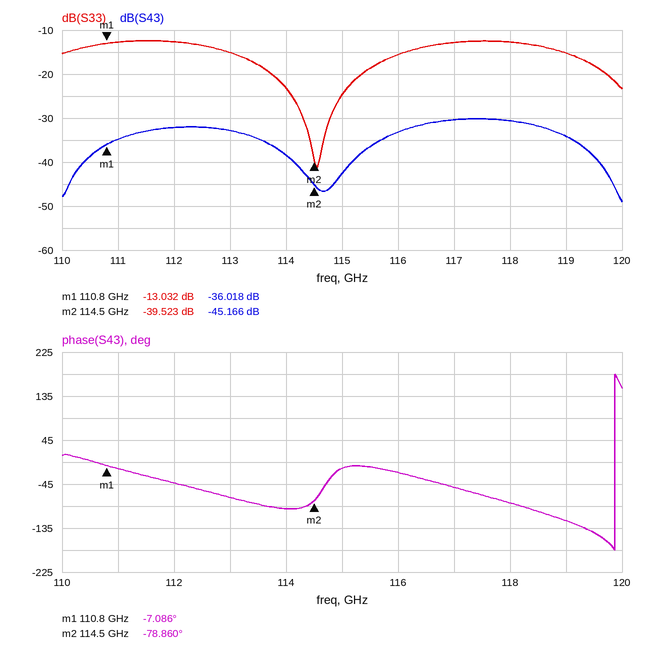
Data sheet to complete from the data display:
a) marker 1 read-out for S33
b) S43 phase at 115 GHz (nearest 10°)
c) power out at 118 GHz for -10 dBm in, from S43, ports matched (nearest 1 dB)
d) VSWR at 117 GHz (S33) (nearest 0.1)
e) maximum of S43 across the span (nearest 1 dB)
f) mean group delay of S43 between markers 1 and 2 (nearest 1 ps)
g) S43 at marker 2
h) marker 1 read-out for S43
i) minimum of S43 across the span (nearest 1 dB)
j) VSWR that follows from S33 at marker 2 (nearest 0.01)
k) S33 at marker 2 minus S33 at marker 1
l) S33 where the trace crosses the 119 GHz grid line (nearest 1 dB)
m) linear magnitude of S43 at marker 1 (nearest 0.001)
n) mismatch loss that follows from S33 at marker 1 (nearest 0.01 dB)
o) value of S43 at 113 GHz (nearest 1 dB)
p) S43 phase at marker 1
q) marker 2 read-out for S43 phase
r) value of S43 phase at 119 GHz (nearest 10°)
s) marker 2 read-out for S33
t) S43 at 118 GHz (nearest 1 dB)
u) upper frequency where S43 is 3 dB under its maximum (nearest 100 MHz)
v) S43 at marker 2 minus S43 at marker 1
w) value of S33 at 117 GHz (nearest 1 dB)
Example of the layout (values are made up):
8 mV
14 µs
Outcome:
-13.032 dB
-10°
-41 dBm
1.6
-30 dB
54 ps
-45.166 dB
-36.018 dB
-49 dB
1.02
-26.491 dB
-15 dB
0.016
0.22 dB
-33 dB
-7.086°
-78.860°
-120°
-39.523 dB
-31 dB
118.8 GHz
-9.148 dB
-13 dB
